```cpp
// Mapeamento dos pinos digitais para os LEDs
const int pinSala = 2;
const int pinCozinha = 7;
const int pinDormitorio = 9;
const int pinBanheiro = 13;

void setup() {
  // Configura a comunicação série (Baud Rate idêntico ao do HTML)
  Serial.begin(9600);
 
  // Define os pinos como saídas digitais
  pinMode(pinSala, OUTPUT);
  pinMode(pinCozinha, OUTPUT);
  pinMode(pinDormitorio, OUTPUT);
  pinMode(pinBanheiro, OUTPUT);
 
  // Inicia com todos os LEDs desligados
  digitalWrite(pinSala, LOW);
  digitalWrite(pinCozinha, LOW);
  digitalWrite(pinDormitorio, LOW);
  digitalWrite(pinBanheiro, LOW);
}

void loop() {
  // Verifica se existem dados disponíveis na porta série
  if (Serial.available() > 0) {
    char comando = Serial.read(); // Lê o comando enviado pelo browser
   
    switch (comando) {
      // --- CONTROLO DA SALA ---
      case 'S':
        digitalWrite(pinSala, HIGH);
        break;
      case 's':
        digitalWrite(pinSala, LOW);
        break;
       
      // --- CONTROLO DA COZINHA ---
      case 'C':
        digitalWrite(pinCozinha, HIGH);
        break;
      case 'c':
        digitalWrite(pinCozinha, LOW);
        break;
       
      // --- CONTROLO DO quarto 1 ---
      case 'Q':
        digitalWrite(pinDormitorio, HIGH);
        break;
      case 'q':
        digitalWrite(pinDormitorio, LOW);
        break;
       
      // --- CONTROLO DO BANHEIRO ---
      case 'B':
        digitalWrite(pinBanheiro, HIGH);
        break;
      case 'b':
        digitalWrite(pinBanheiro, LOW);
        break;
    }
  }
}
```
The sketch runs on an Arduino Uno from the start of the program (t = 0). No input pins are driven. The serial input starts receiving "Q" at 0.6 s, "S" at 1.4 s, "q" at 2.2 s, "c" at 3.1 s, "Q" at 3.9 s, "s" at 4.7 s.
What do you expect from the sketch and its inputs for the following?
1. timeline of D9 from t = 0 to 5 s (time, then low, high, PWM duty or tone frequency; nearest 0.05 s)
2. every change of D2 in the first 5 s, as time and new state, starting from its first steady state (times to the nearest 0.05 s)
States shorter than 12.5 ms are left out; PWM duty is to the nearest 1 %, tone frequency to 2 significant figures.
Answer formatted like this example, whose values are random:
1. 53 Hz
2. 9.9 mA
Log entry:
1. 0 s low; 0.6 s high; 2.2 s low; 3.9 s high
2. 0 s low; 1.4 s high; 4.7 s low
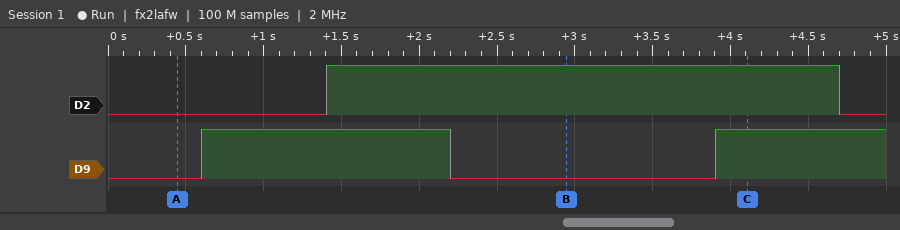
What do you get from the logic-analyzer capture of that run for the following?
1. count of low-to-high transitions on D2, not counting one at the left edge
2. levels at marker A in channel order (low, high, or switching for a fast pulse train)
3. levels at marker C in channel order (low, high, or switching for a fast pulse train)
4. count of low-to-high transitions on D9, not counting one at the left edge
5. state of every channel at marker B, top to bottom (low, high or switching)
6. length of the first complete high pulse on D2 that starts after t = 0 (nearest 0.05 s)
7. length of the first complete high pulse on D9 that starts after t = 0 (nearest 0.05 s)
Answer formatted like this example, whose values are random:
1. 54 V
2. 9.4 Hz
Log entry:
1. 1
2. D2 low, D9 low
3. D2 high, D9 high
4. 2
5. D2 high, D9 low
6. 3.30 s
7. 1.60 s
